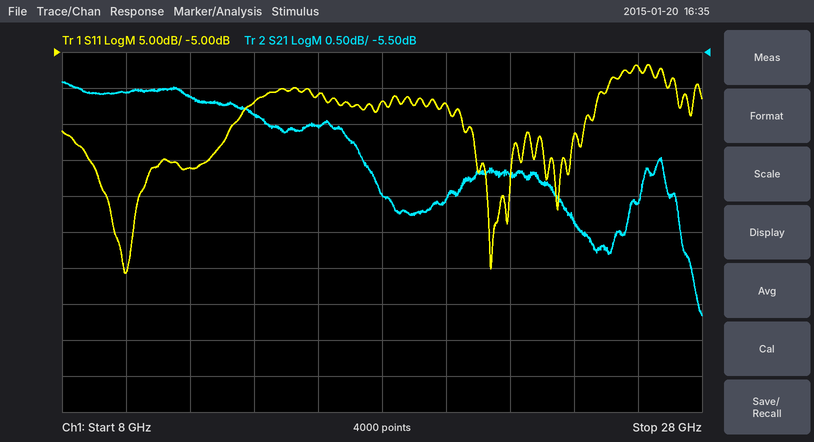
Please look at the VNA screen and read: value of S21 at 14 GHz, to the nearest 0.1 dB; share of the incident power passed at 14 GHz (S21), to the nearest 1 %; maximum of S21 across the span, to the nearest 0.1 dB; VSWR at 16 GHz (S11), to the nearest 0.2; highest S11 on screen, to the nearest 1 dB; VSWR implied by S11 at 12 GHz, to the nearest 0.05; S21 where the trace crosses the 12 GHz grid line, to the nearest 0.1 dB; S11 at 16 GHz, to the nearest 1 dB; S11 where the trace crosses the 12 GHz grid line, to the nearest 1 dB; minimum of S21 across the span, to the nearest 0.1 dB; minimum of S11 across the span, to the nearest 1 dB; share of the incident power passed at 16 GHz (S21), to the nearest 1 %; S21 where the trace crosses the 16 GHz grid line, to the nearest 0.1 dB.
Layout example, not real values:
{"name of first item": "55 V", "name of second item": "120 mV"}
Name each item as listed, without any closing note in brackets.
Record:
{"value of S21 at 14 GHz, to the nearest 0.1 dB": "-6.4 dB", "share of the incident power passed at 14 GHz (S21), to the nearest 1 %": "23 %", "maximum of S21 across the span, to the nearest 0.1 dB": "-5.9 dB", "VSWR at 16 GHz (S11), to the nearest 0.2": "1.8", "highest S11 on screen, to the nearest 1 dB": "-7 dB", "VSWR implied by S11 at 12 GHz, to the nearest 0.05": "1.20", "S21 where the trace crosses the 12 GHz grid line, to the nearest 0.1 dB": "-6.1 dB", "S11 at 16 GHz, to the nearest 1 dB": "-11 dB", "S11 where the trace crosses the 12 GHz grid line, to the nearest 1 dB": "-21 dB", "minimum of S21 across the span, to the nearest 0.1 dB": "-9.2 dB", "minimum of S11 across the span, to the nearest 1 dB": "-36 dB", "share of the incident power passed at 16 GHz (S21), to the nearest 1 %": "22 %", "S21 where the trace crosses the 16 GHz grid line, to the nearest 0.1 dB": "-6.5 dB"}
